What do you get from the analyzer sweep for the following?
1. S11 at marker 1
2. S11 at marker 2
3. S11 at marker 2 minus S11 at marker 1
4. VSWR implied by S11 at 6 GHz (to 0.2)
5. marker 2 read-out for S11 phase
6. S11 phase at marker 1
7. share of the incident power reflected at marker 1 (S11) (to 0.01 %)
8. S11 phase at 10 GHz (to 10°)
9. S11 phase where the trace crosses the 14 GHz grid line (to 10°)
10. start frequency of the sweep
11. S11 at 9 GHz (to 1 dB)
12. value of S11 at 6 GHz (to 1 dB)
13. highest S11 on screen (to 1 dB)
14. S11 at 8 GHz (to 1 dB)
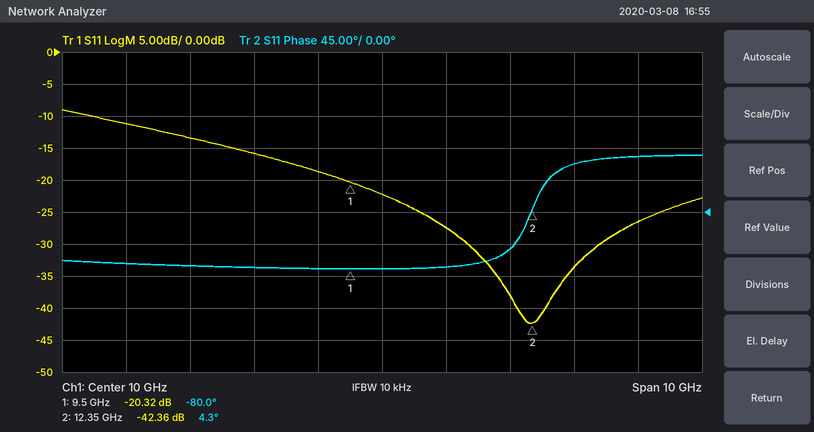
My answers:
-20.32 dB
-42.36 dB
-22.04 dB
1.8
4.3°
-80.0°
0.93 %
-80°
80°
5 GHz
-19 dB
-11 dB
-9 dB
-16 dB
